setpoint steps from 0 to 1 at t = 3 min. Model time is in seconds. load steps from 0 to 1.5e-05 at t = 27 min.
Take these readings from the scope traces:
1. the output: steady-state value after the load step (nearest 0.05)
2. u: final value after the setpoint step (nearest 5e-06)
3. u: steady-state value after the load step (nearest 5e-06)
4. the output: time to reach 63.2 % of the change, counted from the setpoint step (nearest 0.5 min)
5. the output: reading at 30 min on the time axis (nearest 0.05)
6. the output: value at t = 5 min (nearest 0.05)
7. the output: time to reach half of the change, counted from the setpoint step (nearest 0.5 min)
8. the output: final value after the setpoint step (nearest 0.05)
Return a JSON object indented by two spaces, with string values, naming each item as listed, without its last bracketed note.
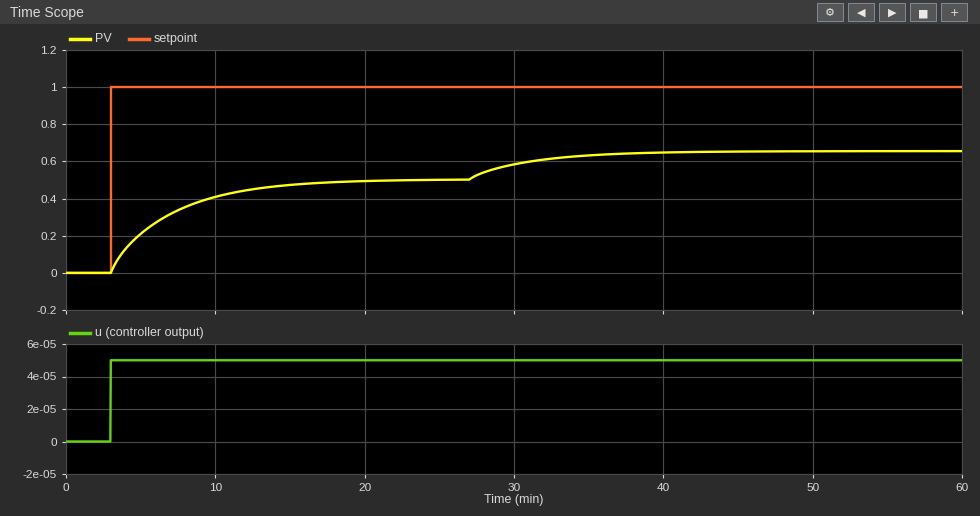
{
  "the output: steady-state value after the load step": "0.65",
  "u: final value after the setpoint step": "0.000050",
  "u: steady-state value after the load step": "0.000050",
  "the output: time to reach 63.2 % of the change, counted from the setpoint step": "4.0 min",
  "the output: reading at 30 min on the time axis": "0.60",
  "the output: value at t = 5 min": "0.20",
  "the output: time to reach half of the change, counted from the setpoint step": "2.5 min",
  "the output: final value after the setpoint step": "0.50"
}
